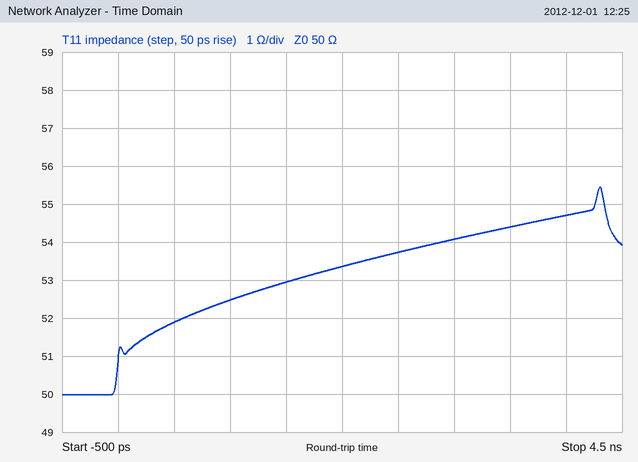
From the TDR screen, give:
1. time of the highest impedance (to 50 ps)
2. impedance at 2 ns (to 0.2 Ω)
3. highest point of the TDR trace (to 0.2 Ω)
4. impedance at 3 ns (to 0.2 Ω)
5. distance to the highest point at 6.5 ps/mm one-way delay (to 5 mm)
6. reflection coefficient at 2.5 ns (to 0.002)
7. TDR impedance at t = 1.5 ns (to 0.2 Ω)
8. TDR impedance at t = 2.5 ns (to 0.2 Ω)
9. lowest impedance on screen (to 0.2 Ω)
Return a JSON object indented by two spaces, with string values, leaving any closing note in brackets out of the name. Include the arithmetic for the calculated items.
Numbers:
{
  "time of the highest impedance": "4.30 ns",
  "impedance at 2 ns": "53.4 Ω",
  "highest point of the TDR trace": "55.4 Ω",
  "impedance at 3 ns": "54.0 Ω",
  "distance to the highest point at 6.5 ps/mm one-way delay": "4.30 ns / 2 / 6.5 ps/mm ≈ 331 mm, so 330 mm to the nearest 5 mm",
  "reflection coefficient at 2.5 ns": "(53.8 − 50)/(53.8 + 50) ≈ +0.0366, so +0.036 to the nearest 0.002",
  "TDR impedance at t = 1.5 ns": "53.0 Ω",
  "TDR impedance at t = 2.5 ns": "53.8 Ω",
  "lowest impedance on screen": "50.0 Ω"
}
